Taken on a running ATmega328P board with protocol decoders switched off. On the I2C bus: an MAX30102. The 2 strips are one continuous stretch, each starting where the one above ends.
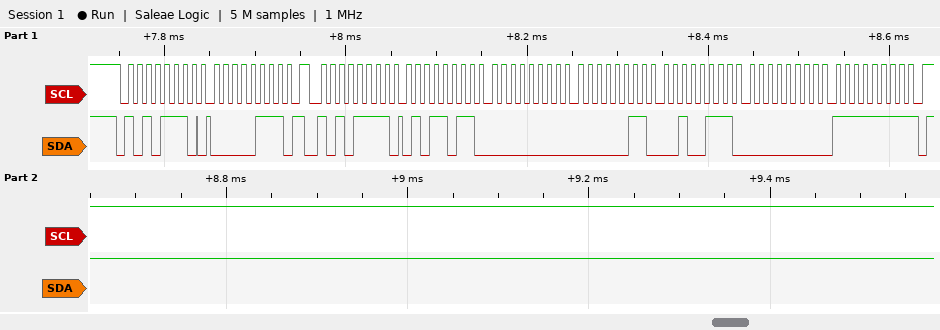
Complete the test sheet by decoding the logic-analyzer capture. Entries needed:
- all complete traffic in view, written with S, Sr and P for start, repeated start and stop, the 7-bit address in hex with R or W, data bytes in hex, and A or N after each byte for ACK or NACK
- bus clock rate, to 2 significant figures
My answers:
S 57W A 07 A Sr 57R A 5B A 00 A 03 A 27 A 00 A FF N P
100 kHz
